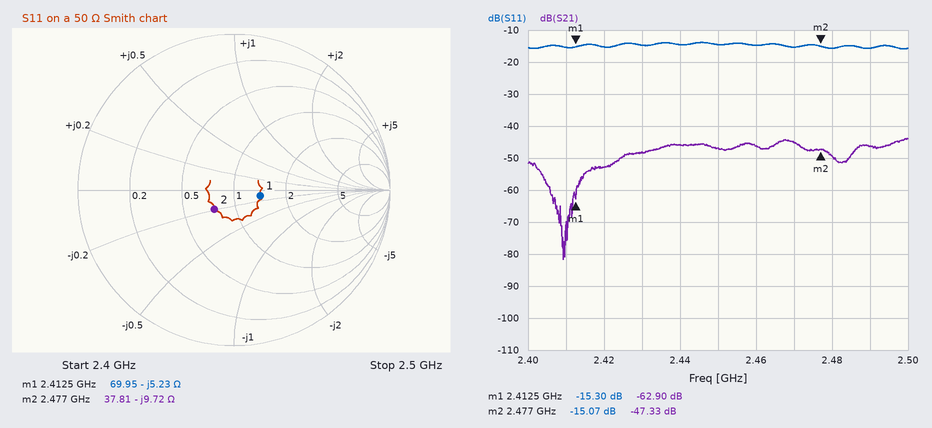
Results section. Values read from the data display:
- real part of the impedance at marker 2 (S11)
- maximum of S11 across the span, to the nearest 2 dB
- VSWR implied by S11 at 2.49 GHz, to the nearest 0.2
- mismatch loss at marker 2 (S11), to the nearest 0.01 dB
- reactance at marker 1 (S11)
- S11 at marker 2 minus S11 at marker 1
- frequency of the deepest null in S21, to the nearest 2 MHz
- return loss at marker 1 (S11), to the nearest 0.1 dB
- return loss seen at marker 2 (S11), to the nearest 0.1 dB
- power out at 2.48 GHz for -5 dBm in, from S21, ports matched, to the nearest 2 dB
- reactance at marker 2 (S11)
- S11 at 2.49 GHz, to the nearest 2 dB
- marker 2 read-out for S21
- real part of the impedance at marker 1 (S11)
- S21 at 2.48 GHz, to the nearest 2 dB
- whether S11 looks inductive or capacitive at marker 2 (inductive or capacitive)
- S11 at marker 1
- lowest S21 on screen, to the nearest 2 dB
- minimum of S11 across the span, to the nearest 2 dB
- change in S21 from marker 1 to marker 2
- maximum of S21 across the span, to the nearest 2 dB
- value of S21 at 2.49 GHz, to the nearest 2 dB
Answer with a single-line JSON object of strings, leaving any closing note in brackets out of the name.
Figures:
{"real part of the impedance at marker 2": "37.81 Ω", "maximum of S11 across the span, to the nearest 2 dB": "-14 dB", "VSWR implied by S11 at 2.49 GHz, to the nearest 0.2": "1.4", "mismatch loss at marker 2 (S11), to the nearest 0.01 dB": "0.14 dB", "reactance at marker 1": "-5.23 Ω", "S11 at marker 2 minus S11 at marker 1": "0.23 dB", "frequency of the deepest null in S21, to the nearest 2 MHz": "2.410 GHz", "return loss at marker 1 (S11), to the nearest 0.1 dB": "15.3 dB", "return loss seen at marker 2 (S11), to the nearest 0.1 dB": "15.1 dB", "power out at 2.48 GHz for -5 dBm in, from S21, ports matched, to the nearest 2 dB": "-54 dBm", "reactance at marker 2": "-9.72 Ω", "S11 at 2.49 GHz, to the nearest 2 dB": "-16 dB", "marker 2 read-out for S21": "-47.33 dB", "real part of the impedance at marker 1": "69.95 Ω", "S21 at 2.48 GHz, to the nearest 2 dB": "-50 dB", "whether S11 looks inductive or capacitive at marker 2": "capacitive", "S11 at marker 1": "-15.30 dB", "lowest S21 on screen, to the nearest 2 dB": "-82 dB", "minimum of S11 across the span, to the nearest 2 dB": "-16 dB", "change in S21 from marker 1 to marker 2": "15.57 dB", "maximum of S21 across the span, to the nearest 2 dB": "-44 dB", "value of S21 at 2.49 GHz, to the nearest 2 dB": "-46 dB"}
